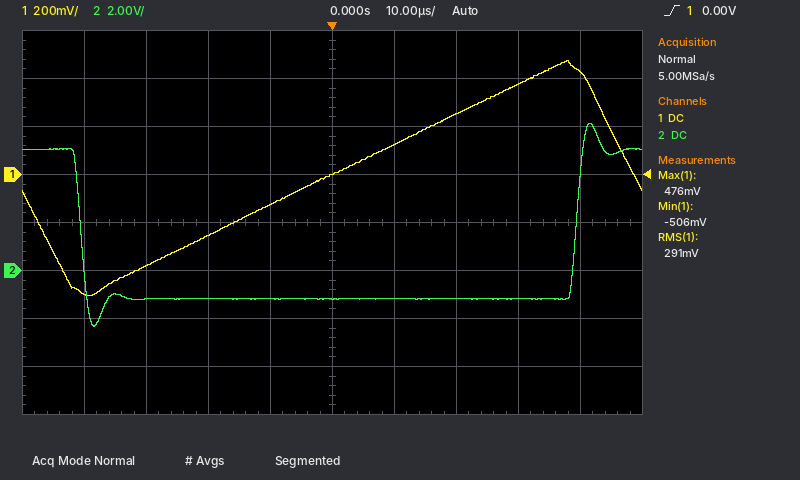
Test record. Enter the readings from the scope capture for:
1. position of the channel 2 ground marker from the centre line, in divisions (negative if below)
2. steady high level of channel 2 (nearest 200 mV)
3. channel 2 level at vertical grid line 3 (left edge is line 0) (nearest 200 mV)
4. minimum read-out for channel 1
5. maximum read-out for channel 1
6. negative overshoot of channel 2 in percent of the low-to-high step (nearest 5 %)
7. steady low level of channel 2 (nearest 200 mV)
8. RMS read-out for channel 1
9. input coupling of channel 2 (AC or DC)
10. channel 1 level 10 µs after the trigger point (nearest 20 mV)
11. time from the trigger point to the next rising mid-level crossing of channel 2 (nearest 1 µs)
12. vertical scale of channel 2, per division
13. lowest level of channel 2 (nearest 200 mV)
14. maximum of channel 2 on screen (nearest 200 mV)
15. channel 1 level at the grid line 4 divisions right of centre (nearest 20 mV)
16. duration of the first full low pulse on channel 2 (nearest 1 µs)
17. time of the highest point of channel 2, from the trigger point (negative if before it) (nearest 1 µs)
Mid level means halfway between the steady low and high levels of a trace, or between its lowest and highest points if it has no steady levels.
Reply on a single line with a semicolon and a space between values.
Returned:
-1.0 div; 5.0 V; -1.2 V; -506 mV; 476 mV; 20 %; -1.2 V; 291 mV; DC; 120 mV; 39 µs; 2 V; -2.4 V; 6.2 V; 420 mV; 80 µs; +42 µs
